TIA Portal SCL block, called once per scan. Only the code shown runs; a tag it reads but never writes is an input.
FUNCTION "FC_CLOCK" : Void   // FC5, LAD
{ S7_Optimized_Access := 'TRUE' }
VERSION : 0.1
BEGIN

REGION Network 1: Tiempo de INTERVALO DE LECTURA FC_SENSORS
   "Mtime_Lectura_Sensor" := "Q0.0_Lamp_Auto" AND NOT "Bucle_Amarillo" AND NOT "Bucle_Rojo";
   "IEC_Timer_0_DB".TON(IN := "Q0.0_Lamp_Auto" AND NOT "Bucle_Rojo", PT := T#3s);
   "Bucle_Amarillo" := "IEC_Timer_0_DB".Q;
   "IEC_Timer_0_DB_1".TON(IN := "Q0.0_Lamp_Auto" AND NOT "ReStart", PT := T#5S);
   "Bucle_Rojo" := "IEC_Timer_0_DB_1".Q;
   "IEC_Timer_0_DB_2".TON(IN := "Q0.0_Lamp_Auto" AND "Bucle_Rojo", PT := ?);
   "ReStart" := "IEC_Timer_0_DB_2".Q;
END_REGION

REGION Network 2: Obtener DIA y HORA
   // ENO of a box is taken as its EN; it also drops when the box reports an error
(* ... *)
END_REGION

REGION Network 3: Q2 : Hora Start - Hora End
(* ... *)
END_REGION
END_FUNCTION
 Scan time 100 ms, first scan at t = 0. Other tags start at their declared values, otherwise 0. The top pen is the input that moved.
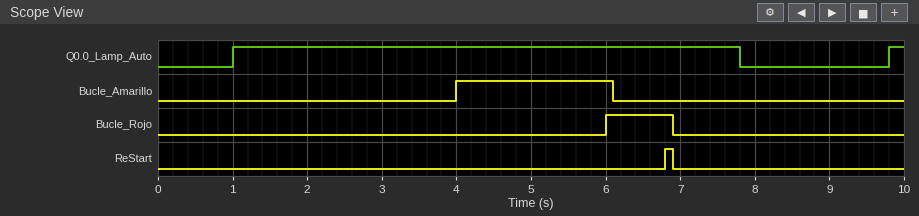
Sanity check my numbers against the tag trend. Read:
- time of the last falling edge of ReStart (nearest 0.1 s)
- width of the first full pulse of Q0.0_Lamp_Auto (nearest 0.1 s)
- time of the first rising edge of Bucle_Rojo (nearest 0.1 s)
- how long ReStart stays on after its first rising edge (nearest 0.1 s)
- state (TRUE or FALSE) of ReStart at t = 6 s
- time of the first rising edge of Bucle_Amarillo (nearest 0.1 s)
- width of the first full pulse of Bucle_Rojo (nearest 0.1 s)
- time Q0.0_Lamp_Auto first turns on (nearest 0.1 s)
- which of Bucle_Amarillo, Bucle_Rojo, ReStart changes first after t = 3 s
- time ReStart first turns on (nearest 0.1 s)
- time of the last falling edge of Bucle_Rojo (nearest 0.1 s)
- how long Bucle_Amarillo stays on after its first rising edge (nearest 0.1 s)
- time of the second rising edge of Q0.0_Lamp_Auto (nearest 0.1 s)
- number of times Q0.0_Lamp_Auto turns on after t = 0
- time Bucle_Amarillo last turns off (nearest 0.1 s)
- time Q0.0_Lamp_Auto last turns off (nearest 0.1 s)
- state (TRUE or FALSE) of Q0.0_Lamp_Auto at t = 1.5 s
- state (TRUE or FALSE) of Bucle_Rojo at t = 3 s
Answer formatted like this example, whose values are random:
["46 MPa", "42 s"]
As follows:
["6.9 s", "6.8 s", "6.0 s", "0.1 s", "FALSE", "4.0 s", "0.9 s", "1.0 s", "Bucle_Amarillo", "6.8 s", "6.9 s", "2.1 s", "9.8 s", "2", "6.1 s", "7.8 s", "TRUE", "FALSE"]
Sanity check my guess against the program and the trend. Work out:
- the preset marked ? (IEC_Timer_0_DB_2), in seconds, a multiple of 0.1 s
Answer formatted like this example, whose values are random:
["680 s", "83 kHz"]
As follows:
["0.8 s"]
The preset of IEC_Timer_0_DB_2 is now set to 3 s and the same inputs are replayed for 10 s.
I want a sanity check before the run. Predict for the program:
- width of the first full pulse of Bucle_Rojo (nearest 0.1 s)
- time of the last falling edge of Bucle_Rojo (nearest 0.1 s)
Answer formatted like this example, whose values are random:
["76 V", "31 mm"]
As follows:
["1.8 s", "7.8 s"]
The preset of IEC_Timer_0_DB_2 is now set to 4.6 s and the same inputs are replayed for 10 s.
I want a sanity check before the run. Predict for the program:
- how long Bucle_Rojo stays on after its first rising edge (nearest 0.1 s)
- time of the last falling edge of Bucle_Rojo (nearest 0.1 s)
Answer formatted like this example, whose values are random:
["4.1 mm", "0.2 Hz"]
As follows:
["1.8 s", "7.8 s"]
